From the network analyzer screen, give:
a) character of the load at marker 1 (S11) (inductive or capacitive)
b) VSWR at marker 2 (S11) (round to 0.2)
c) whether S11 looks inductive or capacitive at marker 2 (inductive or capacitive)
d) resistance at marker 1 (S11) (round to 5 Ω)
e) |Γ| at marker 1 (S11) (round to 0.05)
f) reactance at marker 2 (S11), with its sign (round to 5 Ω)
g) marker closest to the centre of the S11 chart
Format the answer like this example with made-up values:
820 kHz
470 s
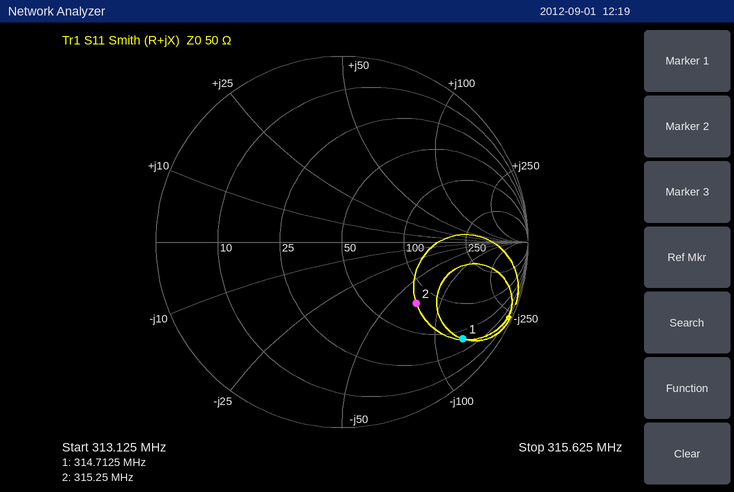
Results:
capacitive
3.2
capacitive
40 Ω
0.85
-70 Ω
marker 2
